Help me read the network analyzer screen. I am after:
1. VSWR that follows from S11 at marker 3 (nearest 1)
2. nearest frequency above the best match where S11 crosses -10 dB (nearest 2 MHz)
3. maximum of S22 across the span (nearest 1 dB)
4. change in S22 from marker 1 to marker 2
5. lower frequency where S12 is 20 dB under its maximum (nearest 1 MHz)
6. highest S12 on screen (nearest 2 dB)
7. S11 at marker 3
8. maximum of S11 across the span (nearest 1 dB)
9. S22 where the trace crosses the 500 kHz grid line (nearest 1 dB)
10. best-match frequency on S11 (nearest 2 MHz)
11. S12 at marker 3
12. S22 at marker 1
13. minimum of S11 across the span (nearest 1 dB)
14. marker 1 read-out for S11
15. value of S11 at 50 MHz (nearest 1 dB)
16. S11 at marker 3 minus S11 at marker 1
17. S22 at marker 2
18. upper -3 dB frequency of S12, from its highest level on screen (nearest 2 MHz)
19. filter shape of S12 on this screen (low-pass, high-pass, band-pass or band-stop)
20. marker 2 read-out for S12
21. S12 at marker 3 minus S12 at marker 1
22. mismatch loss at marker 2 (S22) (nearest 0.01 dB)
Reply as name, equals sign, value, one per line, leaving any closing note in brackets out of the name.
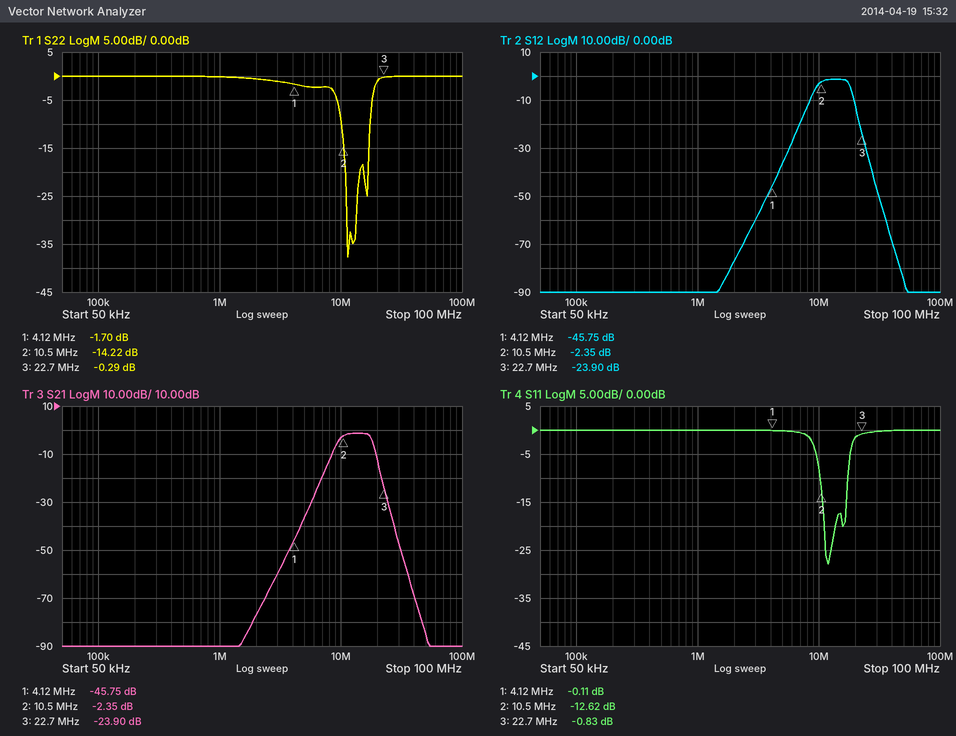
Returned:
VSWR that follows from S11 at marker 3 = 21
nearest frequency above the best match where S11 crosses -10 dB = 18 MHz
maximum of S22 across the span = 0 dB
change in S22 from marker 1 to marker 2 = -12.52 dB
lower frequency where S12 is 20 dB under its maximum = 7 MHz
highest S12 on screen = -2 dB
S11 at marker 3 = -0.83 dB
maximum of S11 across the span = 0 dB
S22 where the trace crosses the 500 kHz grid line = 0 dB
best-match frequency on S11 = 12 MHz
S12 at marker 3 = -23.90 dB
S22 at marker 1 = -1.70 dB
minimum of S11 across the span = -28 dB
marker 1 read-out for S11 = -0.11 dB
value of S11 at 50 MHz = 0 dB
S11 at marker 3 minus S11 at marker 1 = -0.72 dB
S22 at marker 2 = -14.22 dB
upper -3 dB frequency of S12, from its highest level on screen = 18 MHz
filter shape of S12 on this screen = band-pass
marker 2 read-out for S12 = -2.35 dB
S12 at marker 3 minus S12 at marker 1 = 21.85 dB
mismatch loss at marker 2 (S22) = 0.17 dB
